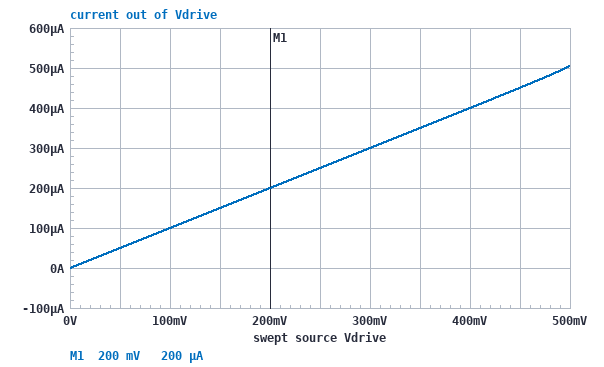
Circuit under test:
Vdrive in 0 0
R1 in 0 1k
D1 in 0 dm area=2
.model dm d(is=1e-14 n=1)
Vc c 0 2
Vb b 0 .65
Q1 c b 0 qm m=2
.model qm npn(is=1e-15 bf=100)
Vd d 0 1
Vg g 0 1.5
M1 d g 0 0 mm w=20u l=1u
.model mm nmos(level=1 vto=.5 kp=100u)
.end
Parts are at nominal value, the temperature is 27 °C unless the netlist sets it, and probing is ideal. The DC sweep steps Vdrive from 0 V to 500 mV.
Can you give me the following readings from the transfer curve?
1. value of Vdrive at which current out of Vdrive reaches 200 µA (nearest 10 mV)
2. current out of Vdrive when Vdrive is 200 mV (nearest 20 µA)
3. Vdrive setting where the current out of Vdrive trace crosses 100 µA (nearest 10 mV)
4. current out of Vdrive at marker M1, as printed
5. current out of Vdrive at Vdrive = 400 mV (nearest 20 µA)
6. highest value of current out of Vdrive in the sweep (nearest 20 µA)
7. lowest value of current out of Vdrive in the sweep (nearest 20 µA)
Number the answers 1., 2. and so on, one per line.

1. 200 mV
2. 200 µA
3. 100 mV
4. 200 µA
5. 400 µA
6. 500 µA
7. 0 A
